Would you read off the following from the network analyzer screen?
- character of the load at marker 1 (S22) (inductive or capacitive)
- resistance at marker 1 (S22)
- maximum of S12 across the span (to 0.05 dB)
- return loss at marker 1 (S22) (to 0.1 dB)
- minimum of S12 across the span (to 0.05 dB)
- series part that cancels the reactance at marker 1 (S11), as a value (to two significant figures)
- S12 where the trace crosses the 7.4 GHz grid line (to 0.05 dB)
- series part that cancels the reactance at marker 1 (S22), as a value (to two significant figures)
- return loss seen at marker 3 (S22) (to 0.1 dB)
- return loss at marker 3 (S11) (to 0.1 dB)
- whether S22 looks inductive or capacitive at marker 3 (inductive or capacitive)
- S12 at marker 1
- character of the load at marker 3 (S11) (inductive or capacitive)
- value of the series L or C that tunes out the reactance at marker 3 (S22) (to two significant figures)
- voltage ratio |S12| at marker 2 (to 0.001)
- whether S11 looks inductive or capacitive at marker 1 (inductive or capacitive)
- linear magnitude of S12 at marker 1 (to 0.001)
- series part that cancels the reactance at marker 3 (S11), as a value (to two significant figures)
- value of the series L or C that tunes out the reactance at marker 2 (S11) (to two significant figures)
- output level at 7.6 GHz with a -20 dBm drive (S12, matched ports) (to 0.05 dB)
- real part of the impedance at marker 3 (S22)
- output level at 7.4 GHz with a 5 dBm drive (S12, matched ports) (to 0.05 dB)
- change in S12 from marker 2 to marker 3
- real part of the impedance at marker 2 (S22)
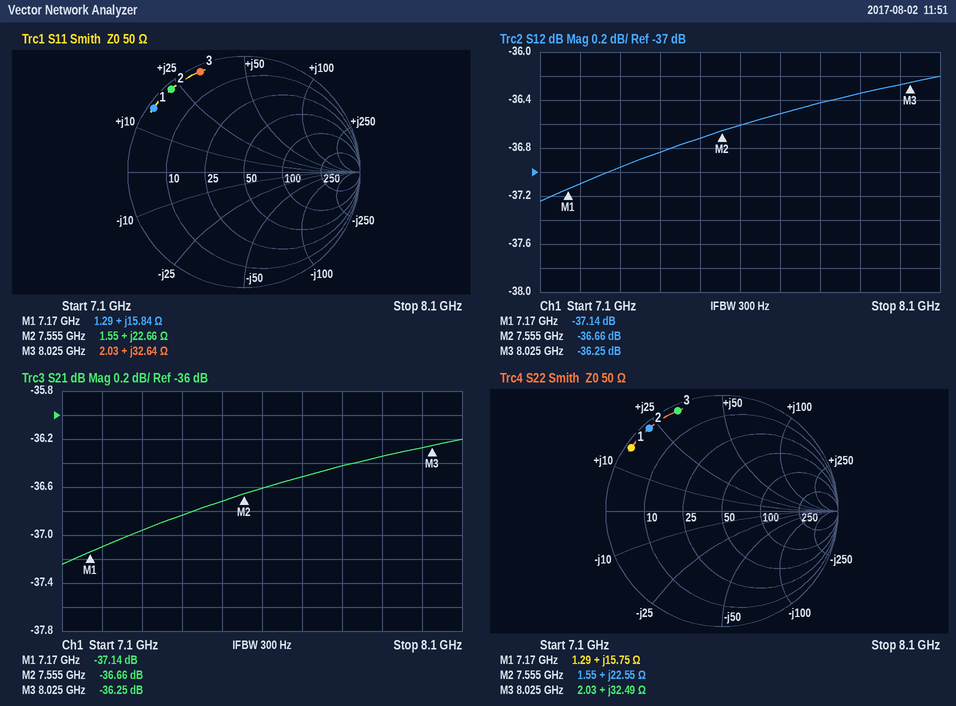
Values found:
inductive
1.29 Ω
-36.20 dB
0.4 dB
-37.25 dB
1.4 pF
-36.85 dB
1.4 pF
0.5 dB
0.5 dB
inductive
-37.14 dB
inductive
610 fF
0.015
inductive
0.014
610 fF
930 fF
-56.60 dBm
2.03 Ω
-31.85 dBm
0.41 dB
1.55 Ω
